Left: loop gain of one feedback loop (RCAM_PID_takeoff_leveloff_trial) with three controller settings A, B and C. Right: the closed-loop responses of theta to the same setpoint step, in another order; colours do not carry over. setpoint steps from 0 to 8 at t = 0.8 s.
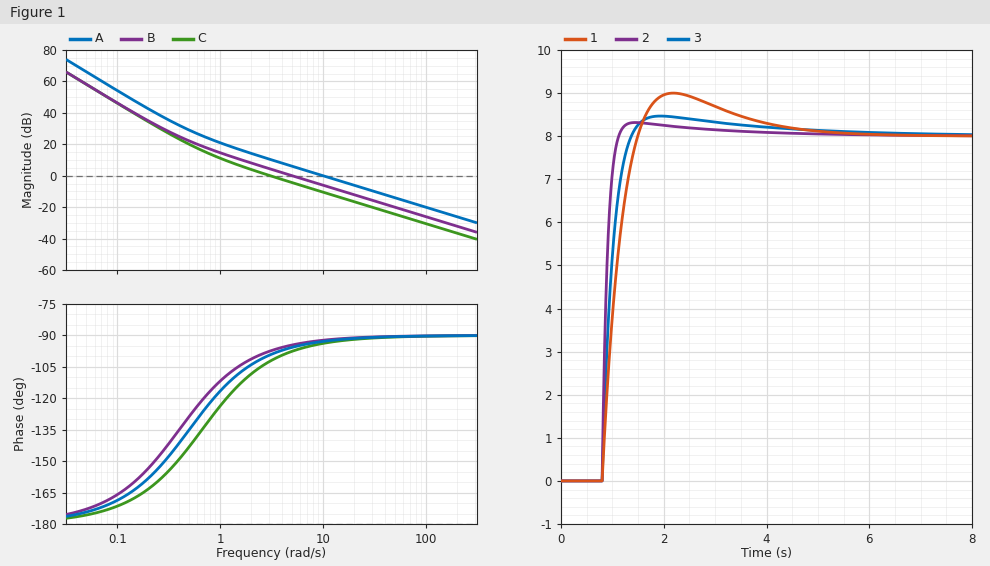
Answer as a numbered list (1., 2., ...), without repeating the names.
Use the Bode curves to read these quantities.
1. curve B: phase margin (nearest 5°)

1. 85°
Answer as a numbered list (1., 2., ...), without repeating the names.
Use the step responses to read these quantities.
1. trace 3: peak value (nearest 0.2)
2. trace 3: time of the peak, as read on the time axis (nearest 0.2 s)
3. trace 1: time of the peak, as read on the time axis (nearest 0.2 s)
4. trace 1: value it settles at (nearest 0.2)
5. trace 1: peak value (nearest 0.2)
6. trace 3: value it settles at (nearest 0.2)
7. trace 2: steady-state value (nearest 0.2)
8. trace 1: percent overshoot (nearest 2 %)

1. 8.4
2. 2.0 s
3. 2.2 s
4. 8.0
5. 9.0
6. 8.0
7. 8.0
8. 12 %
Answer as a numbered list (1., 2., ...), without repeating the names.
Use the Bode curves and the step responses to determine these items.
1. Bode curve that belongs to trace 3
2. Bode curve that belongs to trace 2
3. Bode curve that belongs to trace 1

1. B
2. A
3. C
